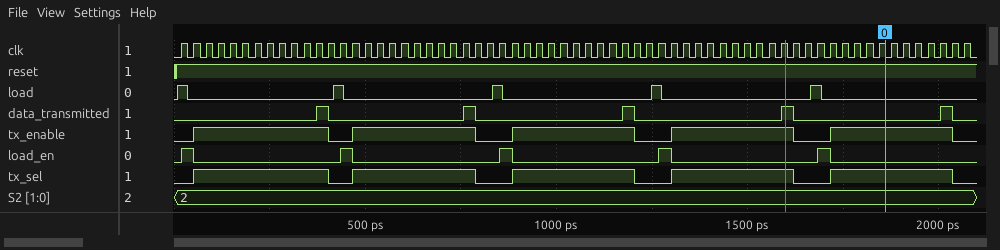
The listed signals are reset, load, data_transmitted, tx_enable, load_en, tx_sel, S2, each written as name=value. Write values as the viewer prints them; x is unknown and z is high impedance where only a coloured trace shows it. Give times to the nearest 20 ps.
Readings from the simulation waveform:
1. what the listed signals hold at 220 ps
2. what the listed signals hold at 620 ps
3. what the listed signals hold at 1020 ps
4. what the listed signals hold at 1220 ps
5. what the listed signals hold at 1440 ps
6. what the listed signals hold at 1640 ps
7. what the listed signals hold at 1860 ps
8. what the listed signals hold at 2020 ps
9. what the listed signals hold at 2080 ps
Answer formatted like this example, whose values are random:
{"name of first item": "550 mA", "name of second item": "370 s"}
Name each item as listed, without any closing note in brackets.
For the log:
{"what the listed signals hold at 220 ps": "reset=1, load=0, data_transmitted=0, tx_enable=1, load_en=0, tx_sel=1, S2=2", "what the listed signals hold at 620 ps": "reset=1, load=0, data_transmitted=0, tx_enable=1, load_en=0, tx_sel=1, S2=2", "what the listed signals hold at 1020 ps": "reset=1, load=0, data_transmitted=0, tx_enable=1, load_en=0, tx_sel=1, S2=2", "what the listed signals hold at 1220 ps": "reset=1, load=0, data_transmitted=0, tx_enable=0, load_en=0, tx_sel=0, S2=2", "what the listed signals hold at 1440 ps": "reset=1, load=0, data_transmitted=0, tx_enable=1, load_en=0, tx_sel=1, S2=2", "what the listed signals hold at 1640 ps": "reset=1, load=0, data_transmitted=0, tx_enable=0, load_en=0, tx_sel=0, S2=2", "what the listed signals hold at 1860 ps": "reset=1, load=0, data_transmitted=0, tx_enable=1, load_en=0, tx_sel=1, S2=2", "what the listed signals hold at 2020 ps": "reset=1, load=0, data_transmitted=1, tx_enable=1, load_en=0, tx_sel=1, S2=2", "what the listed signals hold at 2080 ps": "reset=1, load=0, data_transmitted=0, tx_enable=0, load_en=0, tx_sel=0, S2=2"}
